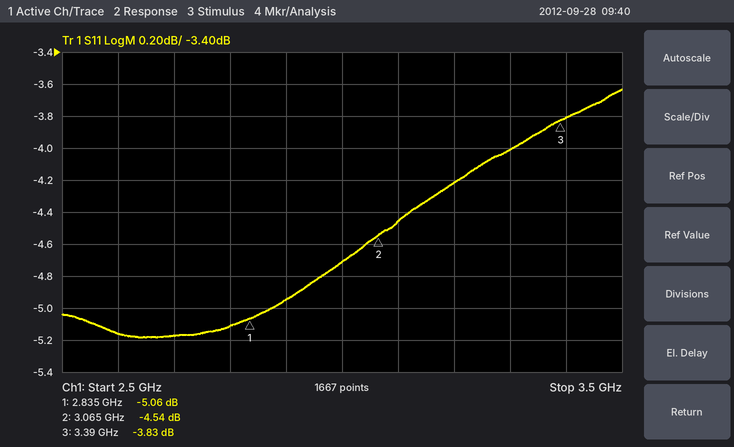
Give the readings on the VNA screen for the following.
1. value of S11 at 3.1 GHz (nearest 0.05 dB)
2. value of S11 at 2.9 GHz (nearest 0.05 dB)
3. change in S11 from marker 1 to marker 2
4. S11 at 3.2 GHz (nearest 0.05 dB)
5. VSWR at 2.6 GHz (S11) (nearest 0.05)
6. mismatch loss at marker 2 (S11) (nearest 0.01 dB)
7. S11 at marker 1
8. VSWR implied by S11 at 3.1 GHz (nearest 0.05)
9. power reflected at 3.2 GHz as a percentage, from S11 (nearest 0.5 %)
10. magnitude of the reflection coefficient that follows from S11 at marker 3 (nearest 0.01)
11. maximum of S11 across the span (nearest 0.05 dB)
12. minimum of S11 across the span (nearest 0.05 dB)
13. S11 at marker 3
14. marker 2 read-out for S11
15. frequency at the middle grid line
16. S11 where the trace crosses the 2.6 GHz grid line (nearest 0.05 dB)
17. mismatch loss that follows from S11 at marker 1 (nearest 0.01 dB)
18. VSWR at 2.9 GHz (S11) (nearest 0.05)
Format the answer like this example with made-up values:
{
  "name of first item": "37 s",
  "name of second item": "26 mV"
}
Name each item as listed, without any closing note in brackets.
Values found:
{
  "value of S11 at 3.1 GHz": "-4.45 dB",
  "value of S11 at 2.9 GHz": "-4.95 dB",
  "change in S11 from marker 1 to marker 2": "0.52 dB",
  "S11 at 3.2 GHz": "-4.20 dB",
  "VSWR at 2.6 GHz (S11)": "3.45",
  "mismatch loss at marker 2 (S11)": "1.88 dB",
  "S11 at marker 1": "-5.06 dB",
  "VSWR implied by S11 at 3.1 GHz": "4.00",
  "power reflected at 3.2 GHz as a percentage, from S11": "38.0 %",
  "magnitude of the reflection coefficient that follows from S11 at marker 3": "0.64",
  "maximum of S11 across the span": "-3.65 dB",
  "minimum of S11 across the span": "-5.20 dB",
  "S11 at marker 3": "-3.83 dB",
  "marker 2 read-out for S11": "-4.54 dB",
  "frequency at the middle grid line": "3 GHz",
  "S11 where the trace crosses the 2.6 GHz grid line": "-5.15 dB",
  "mismatch loss that follows from S11 at marker 1": "1.62 dB",
  "VSWR at 2.9 GHz (S11)": "3.60"
}
